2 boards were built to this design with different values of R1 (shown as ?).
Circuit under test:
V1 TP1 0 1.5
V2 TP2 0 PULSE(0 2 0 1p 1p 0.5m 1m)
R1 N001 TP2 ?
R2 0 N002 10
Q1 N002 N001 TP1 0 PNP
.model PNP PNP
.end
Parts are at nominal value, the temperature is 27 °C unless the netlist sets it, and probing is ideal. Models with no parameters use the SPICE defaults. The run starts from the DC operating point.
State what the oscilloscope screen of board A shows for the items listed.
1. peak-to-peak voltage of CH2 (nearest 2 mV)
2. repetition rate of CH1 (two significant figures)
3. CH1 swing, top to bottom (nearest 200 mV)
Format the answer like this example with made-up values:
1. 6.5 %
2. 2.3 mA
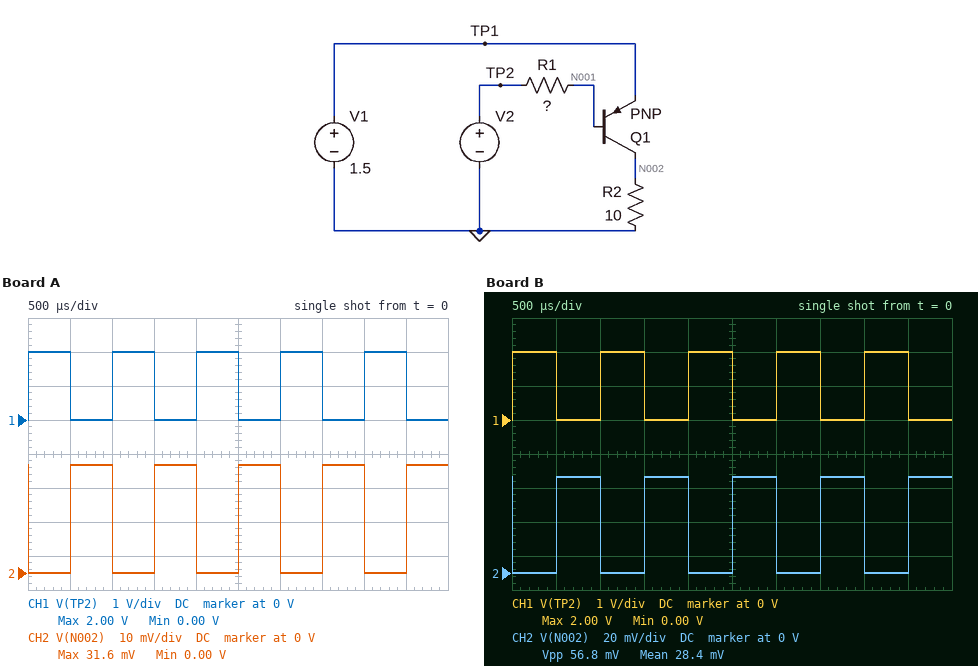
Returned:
1. 32 mV
2. 1.0 kHz
3. 2.0 V
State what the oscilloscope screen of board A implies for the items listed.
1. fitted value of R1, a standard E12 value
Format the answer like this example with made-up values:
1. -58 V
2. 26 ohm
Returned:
1. 22 kΩ
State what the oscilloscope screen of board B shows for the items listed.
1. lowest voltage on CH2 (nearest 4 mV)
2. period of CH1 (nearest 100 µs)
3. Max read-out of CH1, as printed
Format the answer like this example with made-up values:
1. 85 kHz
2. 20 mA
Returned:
1. 0 V
2. 1.0 ms
3. 2.00 V
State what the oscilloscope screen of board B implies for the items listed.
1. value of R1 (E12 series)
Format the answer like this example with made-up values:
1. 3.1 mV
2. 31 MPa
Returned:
1. 12 kΩ
